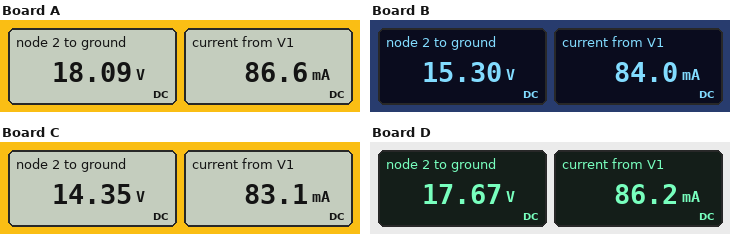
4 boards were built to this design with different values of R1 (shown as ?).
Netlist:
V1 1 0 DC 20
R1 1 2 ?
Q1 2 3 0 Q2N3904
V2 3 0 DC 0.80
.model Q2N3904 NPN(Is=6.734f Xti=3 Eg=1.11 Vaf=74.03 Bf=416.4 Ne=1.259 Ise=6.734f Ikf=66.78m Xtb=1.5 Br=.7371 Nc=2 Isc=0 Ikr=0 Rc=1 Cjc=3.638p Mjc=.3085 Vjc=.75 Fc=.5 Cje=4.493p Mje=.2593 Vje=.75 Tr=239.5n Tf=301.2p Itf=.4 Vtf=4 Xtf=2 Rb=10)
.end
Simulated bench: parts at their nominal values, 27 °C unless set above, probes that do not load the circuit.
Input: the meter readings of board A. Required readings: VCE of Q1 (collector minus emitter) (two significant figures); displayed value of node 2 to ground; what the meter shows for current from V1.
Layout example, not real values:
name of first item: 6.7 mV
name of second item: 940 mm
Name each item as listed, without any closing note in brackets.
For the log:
VCE of Q1 (collector minus emitter): 18 V
displayed value of node 2 to ground: 18.09 V
what the meter shows for current from V1: 86.6 mA
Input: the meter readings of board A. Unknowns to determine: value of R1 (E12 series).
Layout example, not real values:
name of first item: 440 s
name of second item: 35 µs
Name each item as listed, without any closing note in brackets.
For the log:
value of R1: 22 Ω
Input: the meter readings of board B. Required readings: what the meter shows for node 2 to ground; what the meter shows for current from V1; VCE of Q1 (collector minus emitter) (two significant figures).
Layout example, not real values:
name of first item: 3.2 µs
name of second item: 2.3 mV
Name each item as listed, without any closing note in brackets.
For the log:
what the meter shows for node 2 to ground: 15.30 V
what the meter shows for current from V1: 84.0 mA
VCE of Q1 (collector minus emitter): 15 V
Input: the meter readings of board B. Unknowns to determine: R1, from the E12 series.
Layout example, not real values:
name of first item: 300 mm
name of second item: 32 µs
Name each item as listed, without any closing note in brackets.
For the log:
R1, from the E12 series: 56 Ω
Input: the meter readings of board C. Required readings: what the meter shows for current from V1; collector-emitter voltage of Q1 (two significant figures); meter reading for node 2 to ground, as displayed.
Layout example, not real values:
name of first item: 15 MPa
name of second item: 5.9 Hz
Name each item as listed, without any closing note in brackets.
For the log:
what the meter shows for current from V1: 83.1 mA
collector-emitter voltage of Q1: 14 V
meter reading for node 2 to ground, as displayed: 14.35 V
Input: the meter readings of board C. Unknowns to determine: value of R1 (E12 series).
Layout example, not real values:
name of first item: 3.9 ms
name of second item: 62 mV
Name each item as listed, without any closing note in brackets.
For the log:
value of R1: 68 Ω
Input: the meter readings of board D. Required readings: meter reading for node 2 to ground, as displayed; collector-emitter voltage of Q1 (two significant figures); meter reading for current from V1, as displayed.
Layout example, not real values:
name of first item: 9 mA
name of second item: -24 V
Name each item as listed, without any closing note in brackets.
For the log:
meter reading for node 2 to ground, as displayed: 17.67 V
collector-emitter voltage of Q1: 18 V
meter reading for current from V1, as displayed: 86.2 mA
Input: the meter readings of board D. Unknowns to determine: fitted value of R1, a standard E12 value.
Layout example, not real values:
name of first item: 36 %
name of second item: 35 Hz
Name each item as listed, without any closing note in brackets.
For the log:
fitted value of R1, a standard E12 value: 27 Ω
